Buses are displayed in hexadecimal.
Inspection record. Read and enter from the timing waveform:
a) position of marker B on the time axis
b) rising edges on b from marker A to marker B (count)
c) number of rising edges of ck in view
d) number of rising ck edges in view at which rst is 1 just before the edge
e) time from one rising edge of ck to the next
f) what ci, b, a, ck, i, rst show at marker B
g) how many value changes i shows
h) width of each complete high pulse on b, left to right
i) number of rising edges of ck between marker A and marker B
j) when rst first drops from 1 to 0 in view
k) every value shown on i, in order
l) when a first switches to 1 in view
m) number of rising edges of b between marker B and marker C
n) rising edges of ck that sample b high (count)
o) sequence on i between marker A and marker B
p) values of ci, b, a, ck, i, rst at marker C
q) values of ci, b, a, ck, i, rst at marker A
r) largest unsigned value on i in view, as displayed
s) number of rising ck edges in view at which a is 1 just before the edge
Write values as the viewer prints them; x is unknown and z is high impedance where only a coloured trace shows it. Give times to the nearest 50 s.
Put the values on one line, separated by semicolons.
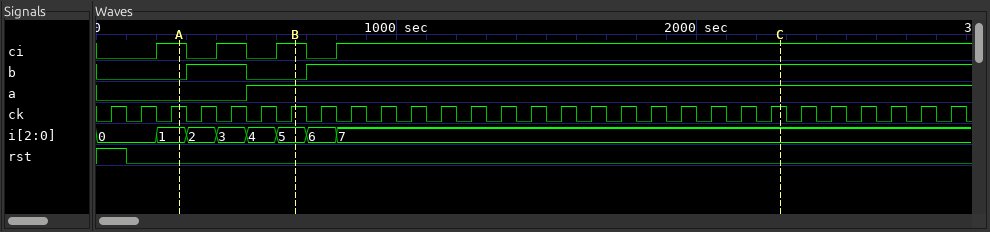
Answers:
650 s; 1; 29; 1; 100 s; ci=1, b=0, a=1, ck=1, i=5, rst=0; 7; 200 s; 4; 100 s; 0, 1, 2, 3, 4, 5, 6, 7; 500 s; 1; 24; 1, 2, 3, 4, 5; ci=1, b=1, a=1, ck=1, i=7, rst=0; ci=1, b=0, a=0, ck=1, i=1, rst=0; 7; 24
